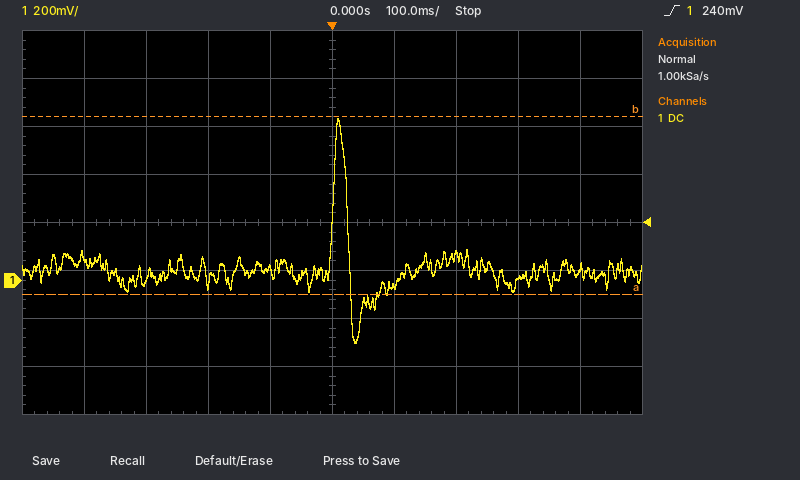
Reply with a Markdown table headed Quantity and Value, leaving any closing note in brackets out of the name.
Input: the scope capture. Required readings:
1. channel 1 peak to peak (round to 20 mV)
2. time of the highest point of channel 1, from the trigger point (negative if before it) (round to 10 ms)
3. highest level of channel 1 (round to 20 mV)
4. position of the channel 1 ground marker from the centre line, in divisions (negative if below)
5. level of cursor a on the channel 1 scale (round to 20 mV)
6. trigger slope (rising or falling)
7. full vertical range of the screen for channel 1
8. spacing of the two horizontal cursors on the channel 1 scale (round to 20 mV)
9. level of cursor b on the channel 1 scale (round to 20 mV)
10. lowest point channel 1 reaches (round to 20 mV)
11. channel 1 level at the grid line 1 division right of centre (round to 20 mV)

| Quantity | Value |
|---|---|
| channel 1 peak to peak | 940 mV |
| time of the highest point of channel 1, from the trigger point (negative if before it) | +10 ms |
| highest level of channel 1 | 680 mV |
| position of the channel 1 ground marker from the centre line, in divisions | -1.2 div |
| level of cursor a on the channel 1 scale | -60 mV |
| trigger slope | rising |
| full vertical range of the screen for channel 1 | 1.6 V |
| spacing of the two horizontal cursors on the channel 1 scale | 740 mV |
| level of cursor b on the channel 1 scale | 680 mV |
| lowest point channel 1 reaches | -260 mV |
| channel 1 level at the grid line 1 division right of centre | -20 mV |
